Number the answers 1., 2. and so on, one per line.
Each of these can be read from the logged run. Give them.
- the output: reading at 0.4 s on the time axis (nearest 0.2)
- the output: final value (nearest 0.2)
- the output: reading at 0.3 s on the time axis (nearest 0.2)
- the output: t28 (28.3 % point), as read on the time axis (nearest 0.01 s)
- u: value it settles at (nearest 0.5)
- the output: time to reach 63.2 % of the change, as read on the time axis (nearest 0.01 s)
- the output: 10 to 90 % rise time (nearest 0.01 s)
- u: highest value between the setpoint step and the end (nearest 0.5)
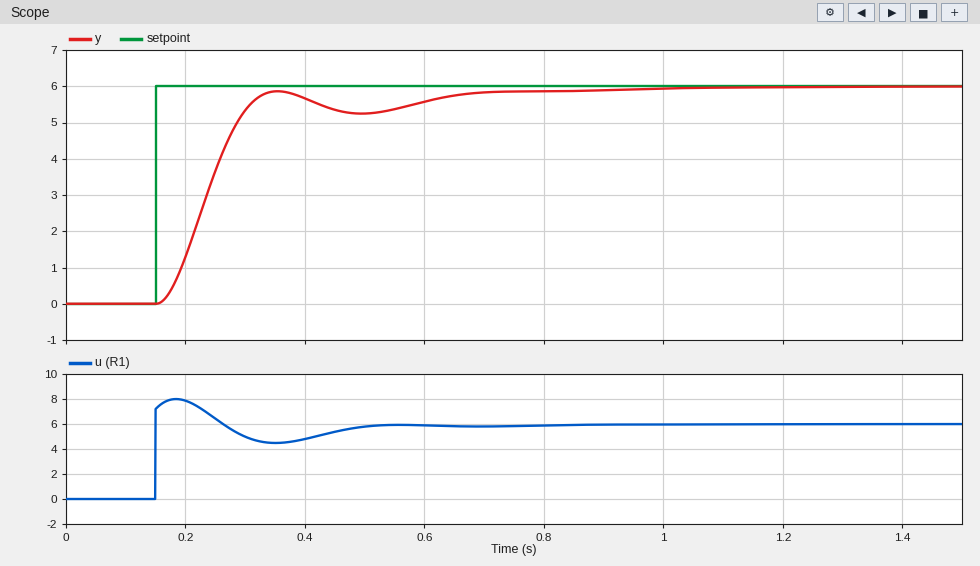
1. 5.6
2. 6.0
3. 5.4
4. 0.21 s
5. 6.0
6. 0.25 s
7. 0.12 s
8. 8.0
